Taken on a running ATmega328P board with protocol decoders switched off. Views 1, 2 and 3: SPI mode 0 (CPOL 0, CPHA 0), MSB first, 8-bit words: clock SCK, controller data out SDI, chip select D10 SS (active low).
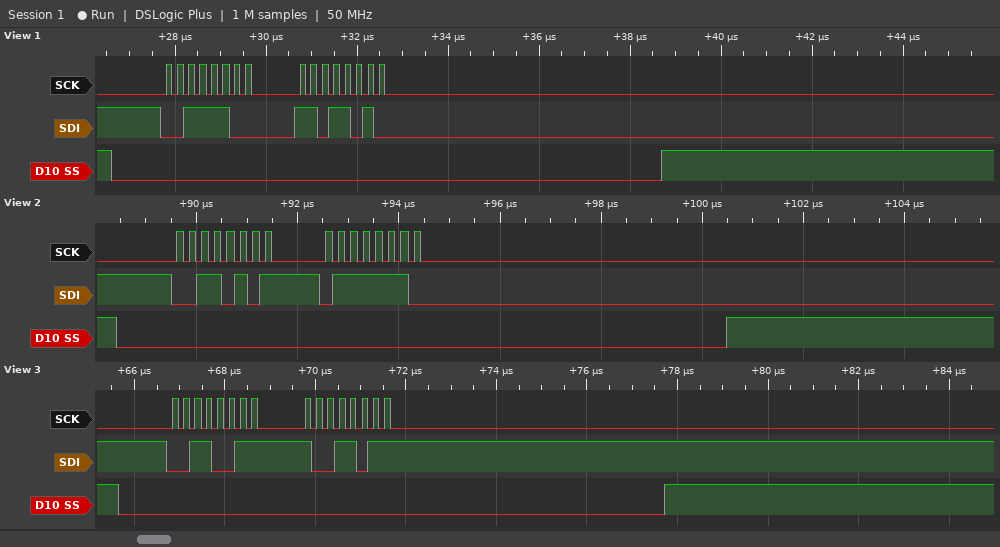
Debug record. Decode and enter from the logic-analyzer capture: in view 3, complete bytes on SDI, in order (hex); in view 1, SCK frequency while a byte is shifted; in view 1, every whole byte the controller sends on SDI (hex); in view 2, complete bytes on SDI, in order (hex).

0x33 0x9B
4 MHz
3C DA
35 7E
